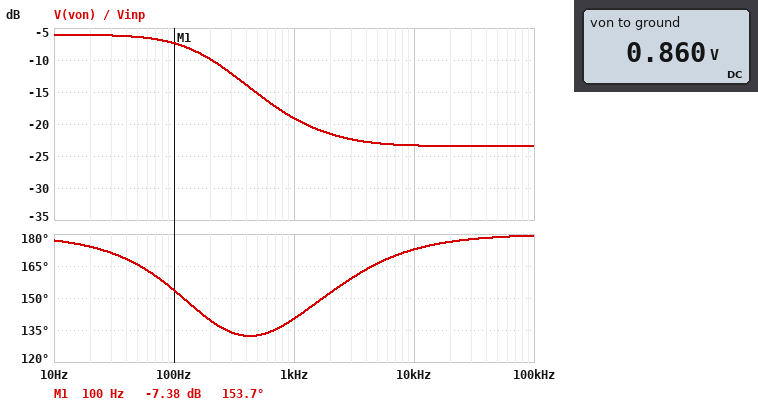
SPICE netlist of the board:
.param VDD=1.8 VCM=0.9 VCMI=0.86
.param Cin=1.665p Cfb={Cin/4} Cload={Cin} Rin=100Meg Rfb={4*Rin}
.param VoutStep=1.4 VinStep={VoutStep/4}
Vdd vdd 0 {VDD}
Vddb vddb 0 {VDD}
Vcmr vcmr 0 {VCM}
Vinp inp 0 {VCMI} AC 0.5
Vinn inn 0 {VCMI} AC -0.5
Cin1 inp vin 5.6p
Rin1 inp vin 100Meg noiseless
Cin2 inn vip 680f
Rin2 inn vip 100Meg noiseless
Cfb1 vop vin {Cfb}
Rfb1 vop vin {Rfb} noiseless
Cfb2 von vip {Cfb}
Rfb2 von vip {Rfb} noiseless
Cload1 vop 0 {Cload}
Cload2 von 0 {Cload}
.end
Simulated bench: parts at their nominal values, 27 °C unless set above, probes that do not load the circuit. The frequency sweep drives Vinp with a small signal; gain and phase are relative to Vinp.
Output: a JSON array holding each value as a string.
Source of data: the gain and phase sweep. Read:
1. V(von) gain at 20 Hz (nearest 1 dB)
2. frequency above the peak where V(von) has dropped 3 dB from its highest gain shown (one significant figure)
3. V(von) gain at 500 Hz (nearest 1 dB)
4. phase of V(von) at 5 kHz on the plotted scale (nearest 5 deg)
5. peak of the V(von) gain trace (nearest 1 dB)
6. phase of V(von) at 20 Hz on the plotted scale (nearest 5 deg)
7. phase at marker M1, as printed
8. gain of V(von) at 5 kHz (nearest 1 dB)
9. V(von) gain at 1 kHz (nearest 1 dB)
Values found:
["-6 dB", "200 Hz", "-15 dB", "165 deg", "-6 dB", "175 deg", "153.7 deg", "-23 dB", "-19 dB"]
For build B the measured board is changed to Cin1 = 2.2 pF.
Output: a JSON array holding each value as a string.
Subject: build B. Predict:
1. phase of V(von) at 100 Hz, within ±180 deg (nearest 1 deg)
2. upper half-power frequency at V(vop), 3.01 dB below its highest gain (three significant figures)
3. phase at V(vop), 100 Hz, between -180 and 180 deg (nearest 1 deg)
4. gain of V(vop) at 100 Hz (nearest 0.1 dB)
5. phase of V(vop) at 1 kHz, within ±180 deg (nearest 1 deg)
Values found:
["154 deg", "163 Hz", "-26 deg", "-1.4 dB", "-33 deg"]
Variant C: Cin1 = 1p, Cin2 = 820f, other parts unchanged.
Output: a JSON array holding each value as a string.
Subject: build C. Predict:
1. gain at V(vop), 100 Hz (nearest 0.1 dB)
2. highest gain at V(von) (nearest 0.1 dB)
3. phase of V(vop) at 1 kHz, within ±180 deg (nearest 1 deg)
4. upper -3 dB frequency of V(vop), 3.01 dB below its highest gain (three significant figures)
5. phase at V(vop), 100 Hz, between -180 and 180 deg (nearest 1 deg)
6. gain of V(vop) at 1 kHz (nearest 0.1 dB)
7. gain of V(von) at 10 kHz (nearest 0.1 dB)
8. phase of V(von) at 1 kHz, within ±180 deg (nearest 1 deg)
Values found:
["-1.4 dB", "-6.0 dB", "-38 deg", "166 Hz", "-26 deg", "-13.1 dB", "-22.9 dB", "141 deg"]
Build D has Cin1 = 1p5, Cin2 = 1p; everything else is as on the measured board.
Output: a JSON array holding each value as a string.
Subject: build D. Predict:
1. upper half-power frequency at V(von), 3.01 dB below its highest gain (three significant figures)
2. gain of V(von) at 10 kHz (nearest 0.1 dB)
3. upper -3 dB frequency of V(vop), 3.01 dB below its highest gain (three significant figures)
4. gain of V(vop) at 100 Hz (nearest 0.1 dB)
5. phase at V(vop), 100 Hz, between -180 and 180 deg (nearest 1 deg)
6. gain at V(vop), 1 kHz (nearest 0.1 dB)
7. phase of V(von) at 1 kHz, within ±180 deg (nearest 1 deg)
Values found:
["166 Hz", "-22.4 dB", "164 Hz", "-1.4 dB", "-26 deg", "-12.9 dB", "142 deg"]
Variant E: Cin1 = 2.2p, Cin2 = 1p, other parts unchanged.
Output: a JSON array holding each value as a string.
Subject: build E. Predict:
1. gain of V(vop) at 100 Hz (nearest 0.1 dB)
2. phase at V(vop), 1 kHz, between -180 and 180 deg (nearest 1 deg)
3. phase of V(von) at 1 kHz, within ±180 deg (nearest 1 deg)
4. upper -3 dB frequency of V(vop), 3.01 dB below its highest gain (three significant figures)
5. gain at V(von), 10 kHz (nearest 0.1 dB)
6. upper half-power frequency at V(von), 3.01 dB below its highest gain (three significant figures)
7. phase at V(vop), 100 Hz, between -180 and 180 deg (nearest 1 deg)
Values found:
["-1.4 dB", "-33 deg", "142 deg", "163 Hz", "-22.4 dB", "166 Hz", "-26 deg"]
